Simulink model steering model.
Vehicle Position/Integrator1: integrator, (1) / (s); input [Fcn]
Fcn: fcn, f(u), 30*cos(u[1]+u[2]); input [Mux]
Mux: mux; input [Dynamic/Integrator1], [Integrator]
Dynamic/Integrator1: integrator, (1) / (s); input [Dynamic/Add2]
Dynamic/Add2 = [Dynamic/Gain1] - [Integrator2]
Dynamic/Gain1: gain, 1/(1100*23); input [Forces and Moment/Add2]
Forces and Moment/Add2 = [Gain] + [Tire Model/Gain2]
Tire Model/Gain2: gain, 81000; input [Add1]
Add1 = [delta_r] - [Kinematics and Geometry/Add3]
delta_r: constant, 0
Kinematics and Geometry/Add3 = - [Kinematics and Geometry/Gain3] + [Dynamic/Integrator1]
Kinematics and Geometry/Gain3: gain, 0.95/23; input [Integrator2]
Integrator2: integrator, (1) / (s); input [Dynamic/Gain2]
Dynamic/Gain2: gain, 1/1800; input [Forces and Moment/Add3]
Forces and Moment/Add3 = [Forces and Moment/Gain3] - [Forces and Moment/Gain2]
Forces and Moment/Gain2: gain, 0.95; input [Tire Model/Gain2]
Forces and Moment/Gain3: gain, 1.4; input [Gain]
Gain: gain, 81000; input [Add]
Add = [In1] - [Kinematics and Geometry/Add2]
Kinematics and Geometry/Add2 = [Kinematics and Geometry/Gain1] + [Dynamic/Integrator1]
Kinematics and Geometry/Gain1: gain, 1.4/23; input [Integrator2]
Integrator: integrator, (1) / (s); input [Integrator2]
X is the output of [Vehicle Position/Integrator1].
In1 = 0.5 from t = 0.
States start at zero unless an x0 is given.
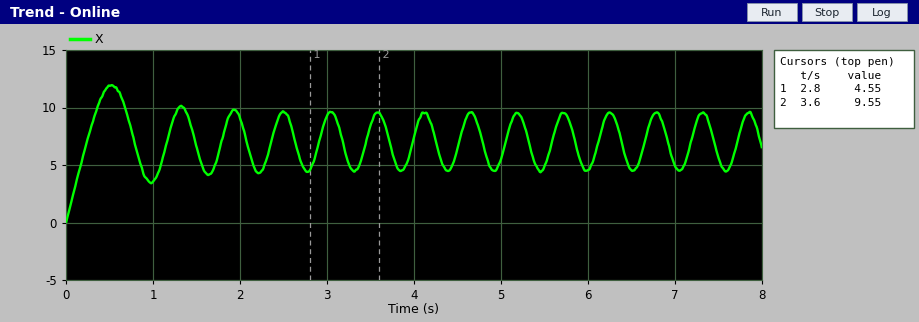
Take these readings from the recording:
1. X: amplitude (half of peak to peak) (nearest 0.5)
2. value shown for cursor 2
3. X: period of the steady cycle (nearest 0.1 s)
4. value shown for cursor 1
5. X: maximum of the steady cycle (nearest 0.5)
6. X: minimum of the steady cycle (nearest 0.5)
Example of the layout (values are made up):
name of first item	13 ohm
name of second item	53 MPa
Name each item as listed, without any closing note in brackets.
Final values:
X: amplitude (half of peak to peak)	2.5
value shown for cursor 2	9.55
X: period of the steady cycle	0.5 s
value shown for cursor 1	4.55
X: maximum of the steady cycle	9.5
X: minimum of the steady cycle	4.5
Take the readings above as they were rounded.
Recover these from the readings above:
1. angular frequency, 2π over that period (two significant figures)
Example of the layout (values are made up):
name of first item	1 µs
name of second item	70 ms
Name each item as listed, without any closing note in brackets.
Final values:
angular frequency, 2π over that period	13 rad/s
